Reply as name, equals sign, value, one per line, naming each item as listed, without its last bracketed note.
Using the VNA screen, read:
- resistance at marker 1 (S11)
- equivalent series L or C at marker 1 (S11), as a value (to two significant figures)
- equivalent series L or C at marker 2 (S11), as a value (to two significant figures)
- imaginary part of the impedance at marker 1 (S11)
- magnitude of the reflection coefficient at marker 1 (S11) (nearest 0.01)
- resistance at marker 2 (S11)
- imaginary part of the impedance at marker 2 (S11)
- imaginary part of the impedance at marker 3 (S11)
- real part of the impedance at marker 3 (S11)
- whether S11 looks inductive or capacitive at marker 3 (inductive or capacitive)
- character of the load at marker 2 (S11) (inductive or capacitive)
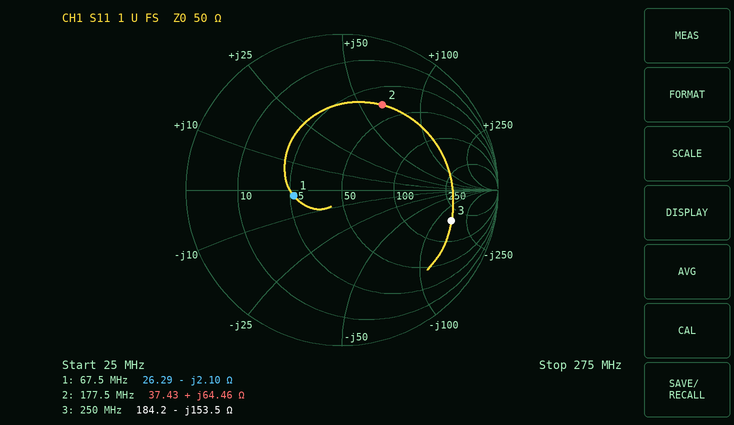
resistance at marker 1 = 26.29 Ω
equivalent series L or C at marker 1 (S11), as a value = 1.1 nF
equivalent series L or C at marker 2 (S11), as a value = 58 nH
imaginary part of the impedance at marker 1 = -2.10 Ω
magnitude of the reflection coefficient at marker 1 (S11) = 0.31
resistance at marker 2 = 37.43 Ω
imaginary part of the impedance at marker 2 = +64.46 Ω
imaginary part of the impedance at marker 3 = -153.5 Ω
real part of the impedance at marker 3 = 184.2 Ω
whether S11 looks inductive or capacitive at marker 3 = capacitive
character of the load at marker 2 (S11) = inductive
